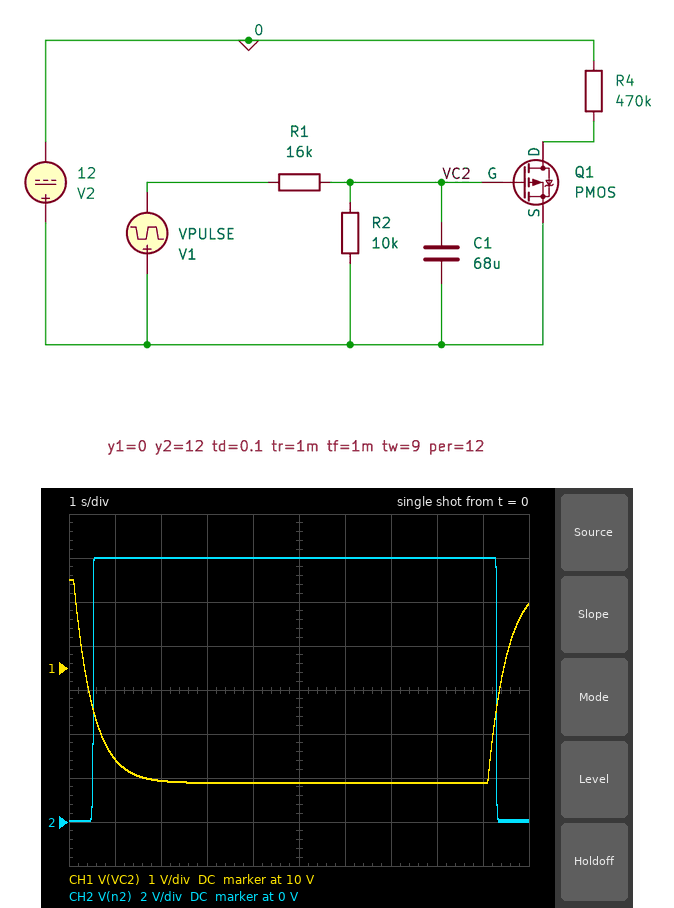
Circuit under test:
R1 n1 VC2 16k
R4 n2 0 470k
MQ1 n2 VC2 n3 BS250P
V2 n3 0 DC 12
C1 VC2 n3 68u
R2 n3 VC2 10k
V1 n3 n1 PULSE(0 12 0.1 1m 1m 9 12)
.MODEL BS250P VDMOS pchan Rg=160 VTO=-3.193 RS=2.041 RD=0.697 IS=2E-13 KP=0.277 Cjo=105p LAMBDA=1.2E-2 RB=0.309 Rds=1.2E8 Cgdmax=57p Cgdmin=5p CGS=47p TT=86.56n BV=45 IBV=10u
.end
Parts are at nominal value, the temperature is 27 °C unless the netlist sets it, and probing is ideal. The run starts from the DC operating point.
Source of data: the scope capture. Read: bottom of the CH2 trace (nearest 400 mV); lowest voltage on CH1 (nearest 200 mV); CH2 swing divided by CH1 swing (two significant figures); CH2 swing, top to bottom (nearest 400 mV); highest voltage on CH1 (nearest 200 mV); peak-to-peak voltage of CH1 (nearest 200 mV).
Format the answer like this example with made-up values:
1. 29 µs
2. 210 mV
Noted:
1. 0 V
2. 7.4 V
3. 2.6
4. 12.0 V
5. 12.0 V
6. 4.6 V
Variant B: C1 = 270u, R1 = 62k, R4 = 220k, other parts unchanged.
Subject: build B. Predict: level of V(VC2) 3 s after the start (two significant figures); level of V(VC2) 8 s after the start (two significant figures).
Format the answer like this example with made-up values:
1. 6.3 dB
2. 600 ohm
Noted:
1. 11 V
2. 10 V
